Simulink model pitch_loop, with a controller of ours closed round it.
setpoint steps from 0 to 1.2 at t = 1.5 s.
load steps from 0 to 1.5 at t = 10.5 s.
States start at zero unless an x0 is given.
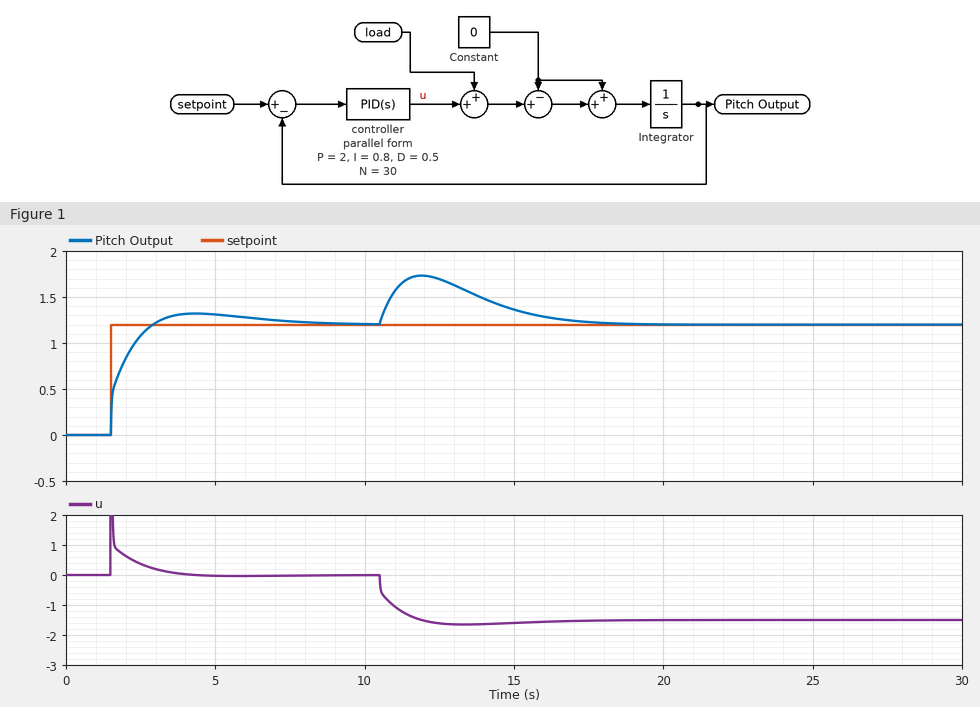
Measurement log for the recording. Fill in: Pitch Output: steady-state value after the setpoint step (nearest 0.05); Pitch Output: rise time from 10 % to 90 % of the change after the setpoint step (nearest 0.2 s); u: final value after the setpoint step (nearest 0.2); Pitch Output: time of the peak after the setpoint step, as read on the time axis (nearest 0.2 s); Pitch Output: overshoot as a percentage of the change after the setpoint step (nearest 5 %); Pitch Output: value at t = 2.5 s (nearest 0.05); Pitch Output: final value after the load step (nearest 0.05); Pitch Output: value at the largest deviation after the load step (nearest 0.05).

1.20
1.0 s
0.0
4.4 s
10 %
1.10
1.20
1.75
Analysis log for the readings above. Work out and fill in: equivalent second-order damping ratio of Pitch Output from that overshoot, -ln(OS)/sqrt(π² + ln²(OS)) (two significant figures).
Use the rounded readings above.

0.59
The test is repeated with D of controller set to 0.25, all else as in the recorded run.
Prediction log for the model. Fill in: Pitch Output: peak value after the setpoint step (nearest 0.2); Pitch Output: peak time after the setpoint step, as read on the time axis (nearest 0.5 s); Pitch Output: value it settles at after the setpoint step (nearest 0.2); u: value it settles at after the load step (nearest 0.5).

1.4
4.0 s
1.2
-1.5
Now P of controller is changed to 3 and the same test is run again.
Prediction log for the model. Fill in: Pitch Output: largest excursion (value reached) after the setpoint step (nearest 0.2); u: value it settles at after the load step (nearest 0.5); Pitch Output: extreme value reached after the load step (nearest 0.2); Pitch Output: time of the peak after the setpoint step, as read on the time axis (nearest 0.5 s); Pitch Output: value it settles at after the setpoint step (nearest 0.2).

1.2
-1.5
1.6
4.0 s
1.2
